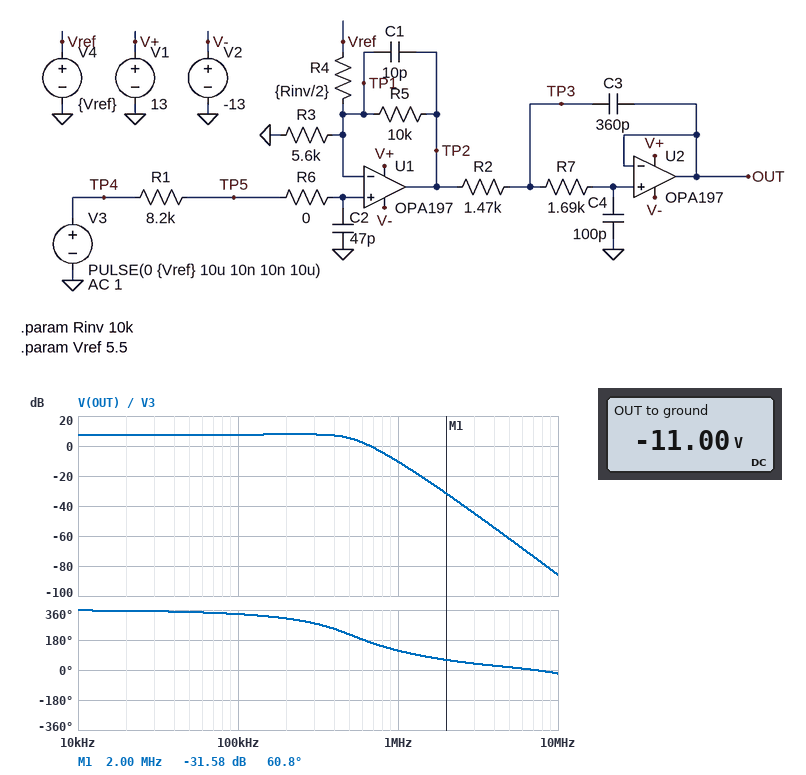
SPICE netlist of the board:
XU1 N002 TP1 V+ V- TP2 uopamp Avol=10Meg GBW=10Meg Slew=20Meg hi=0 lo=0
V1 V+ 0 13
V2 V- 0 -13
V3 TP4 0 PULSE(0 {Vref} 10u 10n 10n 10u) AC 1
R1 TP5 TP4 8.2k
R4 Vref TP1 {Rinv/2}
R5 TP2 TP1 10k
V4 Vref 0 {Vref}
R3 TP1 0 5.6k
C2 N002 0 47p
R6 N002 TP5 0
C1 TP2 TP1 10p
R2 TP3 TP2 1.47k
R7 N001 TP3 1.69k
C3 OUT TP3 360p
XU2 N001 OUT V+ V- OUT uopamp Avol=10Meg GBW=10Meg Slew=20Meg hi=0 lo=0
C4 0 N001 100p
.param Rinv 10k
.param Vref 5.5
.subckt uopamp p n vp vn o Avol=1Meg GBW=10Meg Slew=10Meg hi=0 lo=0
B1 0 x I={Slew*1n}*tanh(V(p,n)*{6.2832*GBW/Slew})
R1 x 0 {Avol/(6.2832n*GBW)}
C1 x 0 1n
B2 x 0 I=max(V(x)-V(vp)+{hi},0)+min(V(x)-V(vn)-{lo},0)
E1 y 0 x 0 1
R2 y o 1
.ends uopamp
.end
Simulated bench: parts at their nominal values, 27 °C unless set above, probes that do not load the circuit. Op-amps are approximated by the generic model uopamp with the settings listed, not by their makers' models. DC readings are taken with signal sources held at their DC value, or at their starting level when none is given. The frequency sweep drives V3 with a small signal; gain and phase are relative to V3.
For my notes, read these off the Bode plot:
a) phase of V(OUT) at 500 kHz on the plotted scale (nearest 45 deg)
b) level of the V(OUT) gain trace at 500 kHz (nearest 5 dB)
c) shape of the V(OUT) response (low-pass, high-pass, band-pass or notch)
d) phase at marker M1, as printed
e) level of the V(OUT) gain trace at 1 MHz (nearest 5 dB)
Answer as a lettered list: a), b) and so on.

a) 225 deg
b) 5 dB
c) low-pass
d) 60.8 deg
e) -10 dB
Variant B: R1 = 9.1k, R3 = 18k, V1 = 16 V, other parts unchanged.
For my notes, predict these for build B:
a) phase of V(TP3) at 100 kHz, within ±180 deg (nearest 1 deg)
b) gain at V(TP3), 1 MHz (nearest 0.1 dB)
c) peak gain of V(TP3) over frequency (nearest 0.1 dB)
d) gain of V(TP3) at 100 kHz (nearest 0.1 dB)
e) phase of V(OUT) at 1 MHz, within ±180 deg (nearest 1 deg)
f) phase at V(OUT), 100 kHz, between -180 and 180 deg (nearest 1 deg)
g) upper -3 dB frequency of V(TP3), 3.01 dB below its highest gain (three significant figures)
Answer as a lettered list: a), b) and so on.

a) -17 deg
b) -10.0 dB
c) 4.7 dB
d) 4.2 dB
e) 123 deg
f) -24 deg
g) 557 kHz
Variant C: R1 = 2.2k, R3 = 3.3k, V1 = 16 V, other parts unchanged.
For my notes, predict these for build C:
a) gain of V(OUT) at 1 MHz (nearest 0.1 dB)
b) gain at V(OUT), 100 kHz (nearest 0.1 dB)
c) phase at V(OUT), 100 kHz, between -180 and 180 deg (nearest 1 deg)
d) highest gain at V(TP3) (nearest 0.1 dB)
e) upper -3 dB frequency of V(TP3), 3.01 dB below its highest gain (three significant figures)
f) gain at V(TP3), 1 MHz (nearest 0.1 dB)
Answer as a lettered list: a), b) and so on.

a) -1.0 dB
b) 15.1 dB
c) -22 deg
d) 15.9 dB
e) 572 kHz
f) 2.3 dB
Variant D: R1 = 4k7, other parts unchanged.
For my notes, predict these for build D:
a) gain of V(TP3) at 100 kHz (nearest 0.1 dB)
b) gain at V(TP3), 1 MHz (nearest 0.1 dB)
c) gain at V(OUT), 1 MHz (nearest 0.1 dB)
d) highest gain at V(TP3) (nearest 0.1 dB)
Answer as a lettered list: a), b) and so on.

a) 12.5 dB
b) -2.3 dB
c) -5.6 dB
d) 13.0 dB
